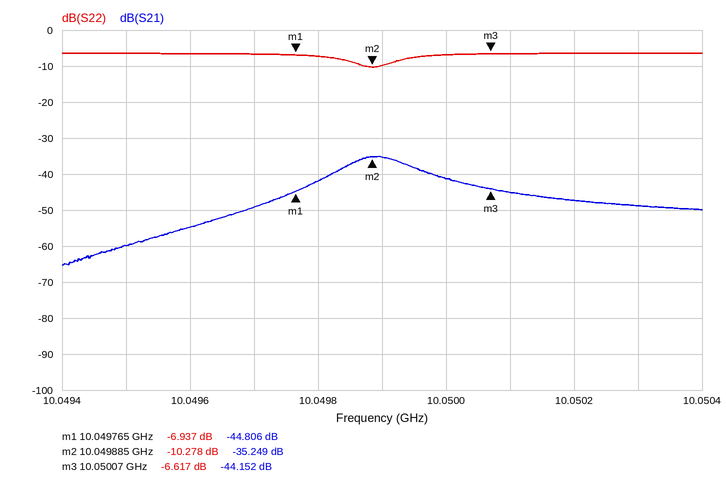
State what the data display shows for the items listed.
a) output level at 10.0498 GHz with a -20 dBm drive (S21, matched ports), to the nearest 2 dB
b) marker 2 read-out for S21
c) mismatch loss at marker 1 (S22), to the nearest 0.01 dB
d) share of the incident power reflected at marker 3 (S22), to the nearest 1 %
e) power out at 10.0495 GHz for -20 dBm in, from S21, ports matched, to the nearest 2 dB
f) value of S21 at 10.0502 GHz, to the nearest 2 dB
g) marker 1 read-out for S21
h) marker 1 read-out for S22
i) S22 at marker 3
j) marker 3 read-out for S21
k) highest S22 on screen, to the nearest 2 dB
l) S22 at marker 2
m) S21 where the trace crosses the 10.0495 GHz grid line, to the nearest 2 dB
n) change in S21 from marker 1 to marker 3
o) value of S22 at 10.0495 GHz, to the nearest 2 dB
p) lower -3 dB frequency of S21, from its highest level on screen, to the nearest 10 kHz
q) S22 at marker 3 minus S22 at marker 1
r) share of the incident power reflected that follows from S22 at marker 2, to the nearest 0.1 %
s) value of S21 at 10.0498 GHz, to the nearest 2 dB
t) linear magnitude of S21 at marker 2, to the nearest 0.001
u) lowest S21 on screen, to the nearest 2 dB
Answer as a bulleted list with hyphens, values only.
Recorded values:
- -62 dBm
- -35.249 dB
- 0.98 dB
- 22 %
- -80 dBm
- -48 dB
- -44.806 dB
- -6.937 dB
- -6.617 dB
- -44.152 dB
- -6 dB
- -10.278 dB
- -60 dB
- 0.654 dB
- -6 dB
- 10.04984 GHz
- 0.320 dB
- 9.4 %
- -42 dB
- 0.017
- -66 dB
